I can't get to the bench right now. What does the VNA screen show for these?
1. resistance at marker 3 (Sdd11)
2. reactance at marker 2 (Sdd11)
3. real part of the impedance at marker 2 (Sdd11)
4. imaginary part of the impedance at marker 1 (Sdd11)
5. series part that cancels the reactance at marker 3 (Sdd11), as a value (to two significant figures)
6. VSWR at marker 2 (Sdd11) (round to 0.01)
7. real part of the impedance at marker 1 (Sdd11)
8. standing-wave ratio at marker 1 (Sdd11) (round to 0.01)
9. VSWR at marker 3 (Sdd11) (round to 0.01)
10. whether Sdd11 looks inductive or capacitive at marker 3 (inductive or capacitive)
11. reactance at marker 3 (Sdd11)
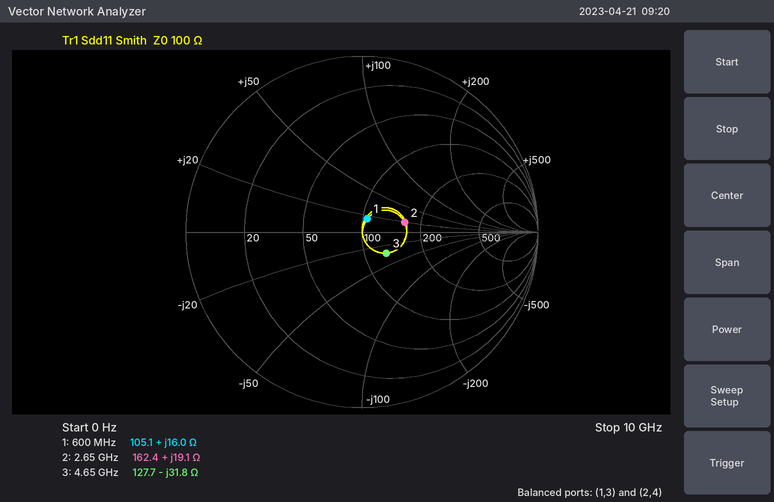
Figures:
127.7 Ω
+19.1 Ω
162.4 Ω
+16.0 Ω
1.1 nH
1.66
105.1 Ω
1.18
1.45
capacitive
-31.8 Ω
